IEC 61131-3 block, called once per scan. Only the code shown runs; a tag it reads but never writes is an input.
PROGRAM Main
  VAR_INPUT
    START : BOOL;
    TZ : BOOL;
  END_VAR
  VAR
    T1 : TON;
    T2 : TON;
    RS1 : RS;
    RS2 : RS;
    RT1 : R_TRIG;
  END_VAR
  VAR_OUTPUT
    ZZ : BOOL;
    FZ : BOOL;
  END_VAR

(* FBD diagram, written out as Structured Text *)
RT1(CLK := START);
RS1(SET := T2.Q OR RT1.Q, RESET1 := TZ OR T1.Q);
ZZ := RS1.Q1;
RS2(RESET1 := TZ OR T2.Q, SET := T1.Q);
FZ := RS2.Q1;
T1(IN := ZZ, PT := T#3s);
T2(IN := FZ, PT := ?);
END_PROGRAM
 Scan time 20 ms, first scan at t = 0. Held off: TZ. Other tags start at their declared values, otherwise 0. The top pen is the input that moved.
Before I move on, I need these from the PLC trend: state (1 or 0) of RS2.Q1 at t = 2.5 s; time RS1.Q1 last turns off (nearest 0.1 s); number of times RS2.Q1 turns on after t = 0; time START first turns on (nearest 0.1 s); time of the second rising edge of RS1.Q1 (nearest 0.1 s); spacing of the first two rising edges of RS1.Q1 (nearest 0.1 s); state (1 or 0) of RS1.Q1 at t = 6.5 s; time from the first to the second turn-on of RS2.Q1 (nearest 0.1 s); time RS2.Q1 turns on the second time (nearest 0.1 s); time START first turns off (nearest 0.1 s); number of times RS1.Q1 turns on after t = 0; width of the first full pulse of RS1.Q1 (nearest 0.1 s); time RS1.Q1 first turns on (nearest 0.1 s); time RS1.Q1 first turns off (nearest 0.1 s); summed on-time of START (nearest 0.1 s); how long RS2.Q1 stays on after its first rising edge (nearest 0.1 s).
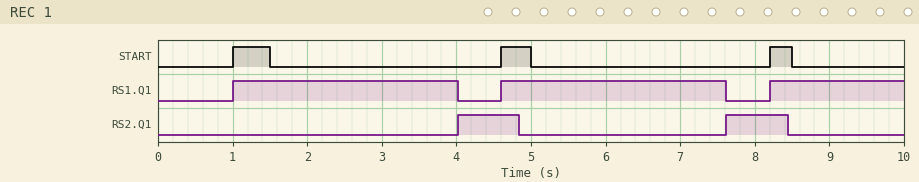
0
7.6 s
2
1.0 s
4.6 s
3.6 s
1
3.6 s
7.6 s
1.5 s
3
3.0 s
1.0 s
4.0 s
1.2 s
0.8 s
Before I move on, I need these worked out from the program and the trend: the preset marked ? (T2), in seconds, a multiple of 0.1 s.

0.8 s
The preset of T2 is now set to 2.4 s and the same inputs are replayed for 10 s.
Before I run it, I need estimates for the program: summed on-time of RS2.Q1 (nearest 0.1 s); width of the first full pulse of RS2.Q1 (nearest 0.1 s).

4.8 s
2.4 s
